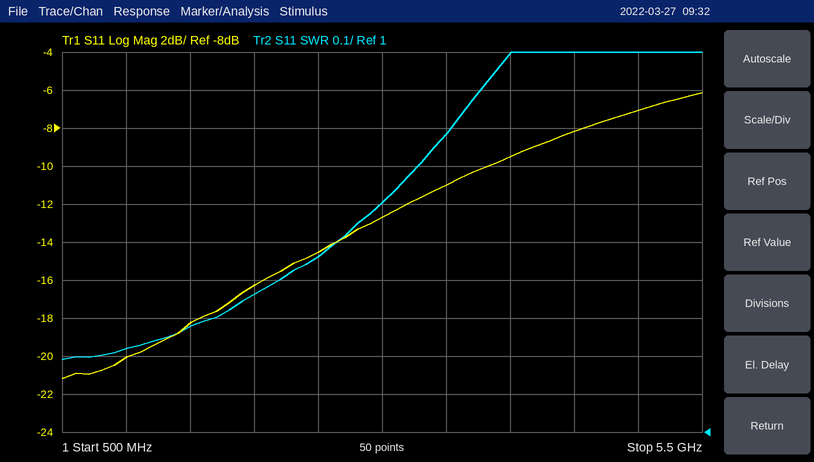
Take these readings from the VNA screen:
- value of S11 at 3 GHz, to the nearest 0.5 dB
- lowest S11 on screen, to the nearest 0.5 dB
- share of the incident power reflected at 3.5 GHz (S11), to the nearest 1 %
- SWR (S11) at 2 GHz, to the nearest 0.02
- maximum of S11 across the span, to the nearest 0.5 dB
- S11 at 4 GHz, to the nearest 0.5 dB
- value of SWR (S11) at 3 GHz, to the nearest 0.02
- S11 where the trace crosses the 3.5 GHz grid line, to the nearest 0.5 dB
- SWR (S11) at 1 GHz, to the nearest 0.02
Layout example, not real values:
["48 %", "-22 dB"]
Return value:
["-12.5 dB", "-21.0 dB", "8 %", "1.36", "-6.0 dB", "-9.5 dB", "1.60", "-11.0 dB", "1.22"]
